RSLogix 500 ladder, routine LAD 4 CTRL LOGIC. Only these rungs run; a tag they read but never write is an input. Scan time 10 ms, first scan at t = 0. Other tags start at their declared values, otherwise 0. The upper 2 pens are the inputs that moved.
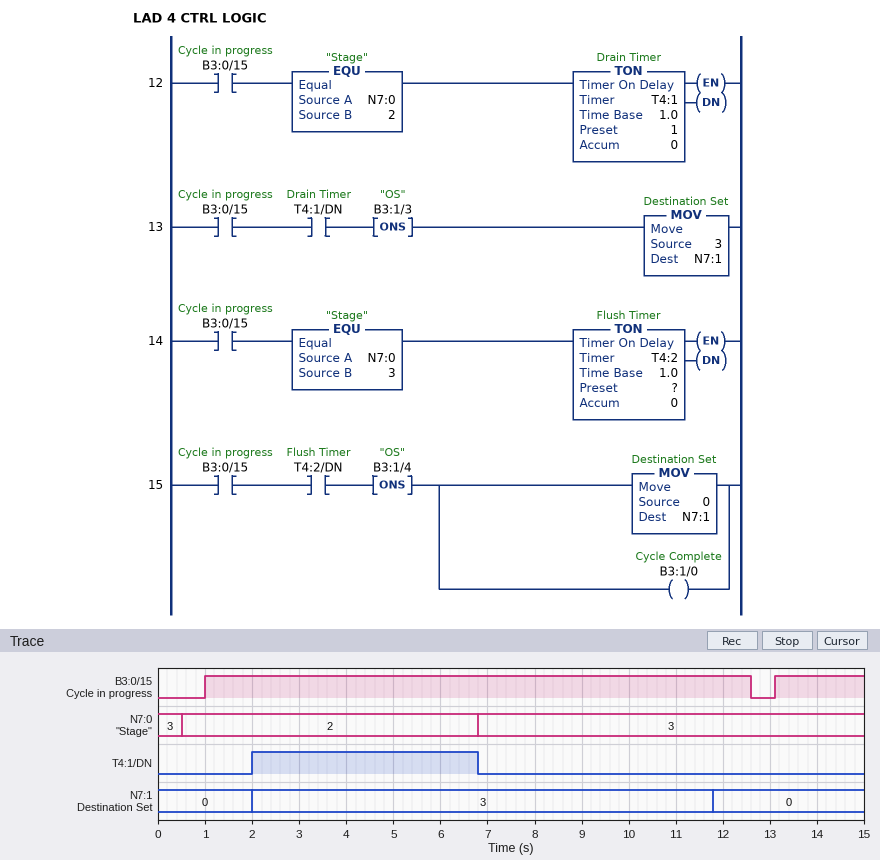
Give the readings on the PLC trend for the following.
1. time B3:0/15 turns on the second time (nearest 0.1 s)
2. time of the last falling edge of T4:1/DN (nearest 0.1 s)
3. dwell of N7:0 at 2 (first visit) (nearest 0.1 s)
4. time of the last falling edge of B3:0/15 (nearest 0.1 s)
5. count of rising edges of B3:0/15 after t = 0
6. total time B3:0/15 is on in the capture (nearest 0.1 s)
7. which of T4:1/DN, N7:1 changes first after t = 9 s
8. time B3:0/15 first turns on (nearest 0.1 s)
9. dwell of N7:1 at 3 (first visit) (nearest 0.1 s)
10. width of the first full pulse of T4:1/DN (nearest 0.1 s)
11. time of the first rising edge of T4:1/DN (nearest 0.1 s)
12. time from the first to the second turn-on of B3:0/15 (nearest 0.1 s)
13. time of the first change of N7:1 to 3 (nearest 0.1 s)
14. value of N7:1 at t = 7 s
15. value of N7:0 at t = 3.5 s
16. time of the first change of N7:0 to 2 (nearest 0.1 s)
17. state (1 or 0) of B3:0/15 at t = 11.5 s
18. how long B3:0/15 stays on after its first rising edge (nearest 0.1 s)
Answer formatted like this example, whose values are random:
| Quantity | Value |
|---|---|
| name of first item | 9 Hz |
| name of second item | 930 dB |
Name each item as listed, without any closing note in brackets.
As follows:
| Quantity | Value |
|---|---|
| time B3:0/15 turns on the second time | 13.1 s |
| time of the last falling edge of T4:1/DN | 6.8 s |
| dwell of N7:0 at 2 (first visit) | 6.3 s |
| time of the last falling edge of B3:0/15 | 12.6 s |
| count of rising edges of B3:0/15 after t = 0 | 2 |
| total time B3:0/15 is on in the capture | 13.5 s |
| which of T4:1/DN, N7:1 changes first after t = 9 s | N7:1 |
| time B3:0/15 first turns on | 1.0 s |
| dwell of N7:1 at 3 (first visit) | 9.8 s |
| width of the first full pulse of T4:1/DN | 4.8 s |
| time of the first rising edge of T4:1/DN | 2.0 s |
| time from the first to the second turn-on of B3:0/15 | 12.1 s |
| time of the first change of N7:1 to 3 | 2.0 s |
| value of N7:1 at t = 7 s | 3 |
| value of N7:0 at t = 3.5 s | 2 |
| time of the first change of N7:0 to 2 | 0.5 s |
| state (1 or 0) of B3:0/15 at t = 11.5 s | 1 |
| how long B3:0/15 stays on after its first rising edge | 11.6 s |
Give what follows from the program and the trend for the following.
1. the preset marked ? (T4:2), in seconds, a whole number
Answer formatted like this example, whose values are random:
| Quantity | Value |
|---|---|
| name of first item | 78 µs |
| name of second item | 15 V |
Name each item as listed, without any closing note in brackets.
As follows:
| Quantity | Value |
|---|---|
| the preset marked ? (T4:2), in seconds, a whole number | 5 s |
